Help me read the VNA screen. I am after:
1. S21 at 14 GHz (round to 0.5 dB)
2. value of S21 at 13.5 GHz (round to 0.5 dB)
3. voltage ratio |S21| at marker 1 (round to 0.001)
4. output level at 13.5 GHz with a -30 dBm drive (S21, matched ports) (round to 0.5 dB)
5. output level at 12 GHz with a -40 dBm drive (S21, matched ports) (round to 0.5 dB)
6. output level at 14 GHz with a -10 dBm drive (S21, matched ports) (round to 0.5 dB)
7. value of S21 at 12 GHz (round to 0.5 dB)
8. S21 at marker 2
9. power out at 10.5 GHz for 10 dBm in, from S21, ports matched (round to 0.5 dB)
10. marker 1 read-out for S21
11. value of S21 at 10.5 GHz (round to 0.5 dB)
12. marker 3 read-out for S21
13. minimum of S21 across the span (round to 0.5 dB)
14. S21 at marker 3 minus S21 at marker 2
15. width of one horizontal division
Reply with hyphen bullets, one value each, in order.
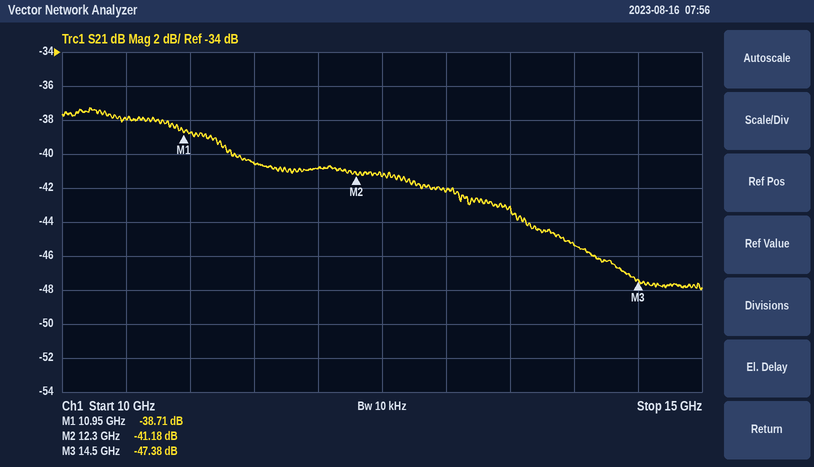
- -45.5 dB
- -43.0 dB
- 0.012
- -73.0 dBm
- -81.0 dBm
- -55.5 dBm
- -41.0 dB
- -41.18 dB
- -28.0 dBm
- -38.71 dB
- -38.0 dB
- -47.38 dB
- -48.0 dB
- -6.20 dB
- 500 MHz
